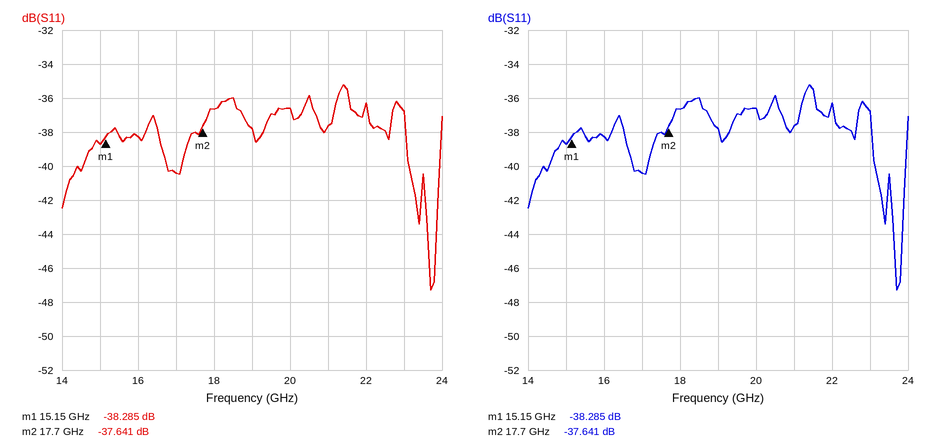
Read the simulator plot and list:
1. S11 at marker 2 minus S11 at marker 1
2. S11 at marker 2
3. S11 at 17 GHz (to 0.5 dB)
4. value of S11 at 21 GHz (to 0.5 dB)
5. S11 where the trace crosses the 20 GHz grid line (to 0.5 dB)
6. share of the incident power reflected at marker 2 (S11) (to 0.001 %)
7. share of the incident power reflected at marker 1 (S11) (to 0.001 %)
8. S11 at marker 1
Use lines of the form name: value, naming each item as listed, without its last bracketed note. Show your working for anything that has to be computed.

S11 at marker 2 minus S11 at marker 1: -37.641 − (-38.285) = 0.644 dB
S11 at marker 2: -37.641 dB
S11 at 17 GHz: -40.5 dB
value of S11 at 21 GHz: -37.5 dB
S11 where the trace crosses the 20 GHz grid line: -36.5 dB
share of the incident power reflected at marker 2 (S11): 10^(-37.641/10) ≈ 0.017 %
share of the incident power reflected at marker 1 (S11): 10^(-38.285/10) ≈ 0.015 %
S11 at marker 1: -38.285 dB
